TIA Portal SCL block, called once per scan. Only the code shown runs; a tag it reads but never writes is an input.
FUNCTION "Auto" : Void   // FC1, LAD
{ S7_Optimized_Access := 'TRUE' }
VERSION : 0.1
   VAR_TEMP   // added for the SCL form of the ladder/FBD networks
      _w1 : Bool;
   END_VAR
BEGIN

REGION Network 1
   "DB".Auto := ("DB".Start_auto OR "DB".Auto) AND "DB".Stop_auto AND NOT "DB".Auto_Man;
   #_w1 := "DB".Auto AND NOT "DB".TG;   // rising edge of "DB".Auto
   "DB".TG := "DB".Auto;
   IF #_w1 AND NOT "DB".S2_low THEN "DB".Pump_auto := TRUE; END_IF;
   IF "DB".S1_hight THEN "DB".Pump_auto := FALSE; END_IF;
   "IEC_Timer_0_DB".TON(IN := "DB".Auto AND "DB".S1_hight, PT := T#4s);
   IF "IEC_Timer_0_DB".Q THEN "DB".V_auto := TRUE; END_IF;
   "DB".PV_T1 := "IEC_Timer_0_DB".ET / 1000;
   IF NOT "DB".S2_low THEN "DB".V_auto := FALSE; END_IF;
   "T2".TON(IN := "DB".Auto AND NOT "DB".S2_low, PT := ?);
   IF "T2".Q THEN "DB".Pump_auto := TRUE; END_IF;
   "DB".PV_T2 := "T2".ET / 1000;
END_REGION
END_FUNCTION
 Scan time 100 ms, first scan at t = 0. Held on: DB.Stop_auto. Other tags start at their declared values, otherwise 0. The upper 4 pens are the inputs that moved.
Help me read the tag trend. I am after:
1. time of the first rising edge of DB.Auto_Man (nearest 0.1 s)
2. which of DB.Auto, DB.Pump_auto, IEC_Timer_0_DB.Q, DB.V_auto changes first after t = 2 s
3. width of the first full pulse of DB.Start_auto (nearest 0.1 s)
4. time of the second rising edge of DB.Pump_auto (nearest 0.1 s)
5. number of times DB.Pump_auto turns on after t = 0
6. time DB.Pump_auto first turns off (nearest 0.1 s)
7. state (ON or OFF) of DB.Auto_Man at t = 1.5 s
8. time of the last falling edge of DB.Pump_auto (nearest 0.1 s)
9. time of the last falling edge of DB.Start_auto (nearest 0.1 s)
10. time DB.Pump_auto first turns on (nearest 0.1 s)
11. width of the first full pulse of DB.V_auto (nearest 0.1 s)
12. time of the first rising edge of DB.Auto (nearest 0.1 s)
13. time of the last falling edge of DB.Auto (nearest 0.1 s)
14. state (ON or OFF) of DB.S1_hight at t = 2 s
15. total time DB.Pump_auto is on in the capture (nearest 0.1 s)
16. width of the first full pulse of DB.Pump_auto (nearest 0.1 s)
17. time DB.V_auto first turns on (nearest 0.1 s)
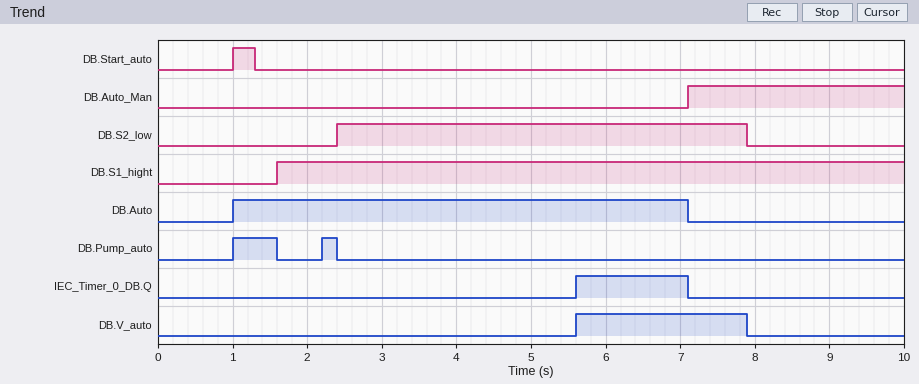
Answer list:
7.1 s
DB.Pump_auto
0.3 s
2.2 s
2
1.6 s
OFF
2.4 s
1.3 s
1.0 s
2.3 s
1.0 s
7.1 s
ON
0.8 s
0.6 s
5.6 s
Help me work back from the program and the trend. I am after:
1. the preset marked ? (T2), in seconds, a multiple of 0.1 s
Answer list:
1.2 s
